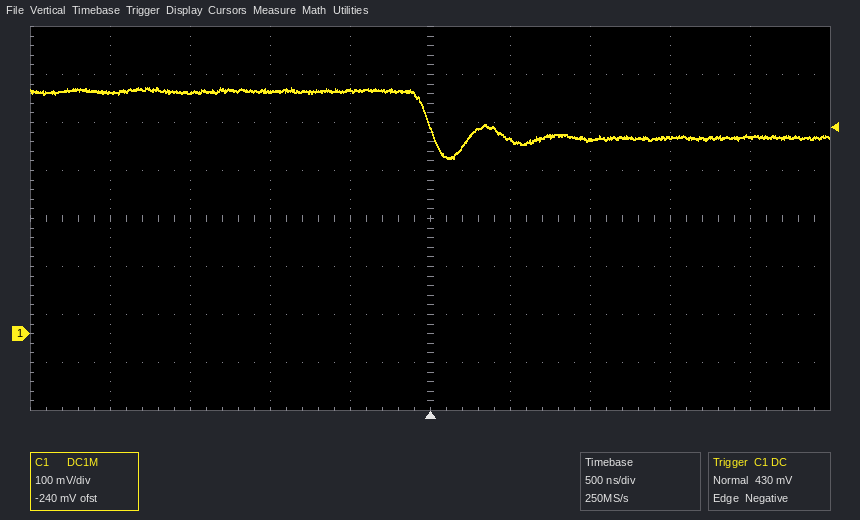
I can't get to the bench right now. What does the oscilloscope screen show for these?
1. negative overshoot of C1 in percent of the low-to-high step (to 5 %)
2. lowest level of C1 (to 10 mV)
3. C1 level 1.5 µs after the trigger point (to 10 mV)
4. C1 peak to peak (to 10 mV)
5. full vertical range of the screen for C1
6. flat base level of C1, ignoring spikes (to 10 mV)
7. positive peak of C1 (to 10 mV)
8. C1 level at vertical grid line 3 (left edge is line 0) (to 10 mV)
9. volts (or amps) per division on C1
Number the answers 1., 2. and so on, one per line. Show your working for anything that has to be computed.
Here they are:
1. 45 %
2. 360 mV
3. 410 mV
4. 510 mV − (360 mV) = 150 mV
5. 800 mV
6. 410 mV
7. 510 mV
8. 500 mV
9. 100 mV
